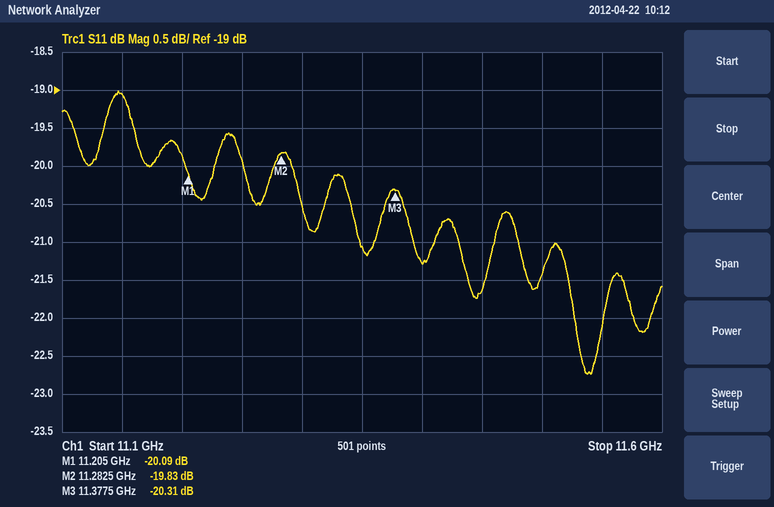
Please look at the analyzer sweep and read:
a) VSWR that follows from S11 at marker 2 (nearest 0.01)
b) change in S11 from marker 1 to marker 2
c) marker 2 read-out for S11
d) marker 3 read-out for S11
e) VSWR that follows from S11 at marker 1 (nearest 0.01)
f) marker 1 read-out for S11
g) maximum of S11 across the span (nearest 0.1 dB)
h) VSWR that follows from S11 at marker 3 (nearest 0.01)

1.23
0.26 dB
-19.83 dB
-20.31 dB
1.22
-20.09 dB
-19.0 dB
1.21
